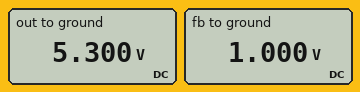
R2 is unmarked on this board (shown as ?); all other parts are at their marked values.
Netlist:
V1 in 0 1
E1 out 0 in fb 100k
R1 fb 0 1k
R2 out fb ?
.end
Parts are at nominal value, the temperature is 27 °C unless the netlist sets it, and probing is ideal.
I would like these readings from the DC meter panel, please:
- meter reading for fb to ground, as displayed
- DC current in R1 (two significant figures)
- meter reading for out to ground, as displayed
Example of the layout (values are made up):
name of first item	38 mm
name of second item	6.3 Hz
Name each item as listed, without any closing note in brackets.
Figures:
meter reading for fb to ground, as displayed	1.000 V
DC current in R1	1.0 mA
meter reading for out to ground, as displayed	5.300 V
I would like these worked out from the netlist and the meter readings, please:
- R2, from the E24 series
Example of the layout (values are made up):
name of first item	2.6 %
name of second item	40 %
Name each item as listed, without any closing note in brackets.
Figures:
R2, from the E24 series	4.3 kΩ
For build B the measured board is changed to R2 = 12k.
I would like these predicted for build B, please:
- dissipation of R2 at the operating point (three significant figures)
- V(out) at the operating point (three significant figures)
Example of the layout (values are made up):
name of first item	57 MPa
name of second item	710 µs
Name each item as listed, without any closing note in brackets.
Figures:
dissipation of R2 at the operating point	12.0 mW
V(out) at the operating point	13.0 V
